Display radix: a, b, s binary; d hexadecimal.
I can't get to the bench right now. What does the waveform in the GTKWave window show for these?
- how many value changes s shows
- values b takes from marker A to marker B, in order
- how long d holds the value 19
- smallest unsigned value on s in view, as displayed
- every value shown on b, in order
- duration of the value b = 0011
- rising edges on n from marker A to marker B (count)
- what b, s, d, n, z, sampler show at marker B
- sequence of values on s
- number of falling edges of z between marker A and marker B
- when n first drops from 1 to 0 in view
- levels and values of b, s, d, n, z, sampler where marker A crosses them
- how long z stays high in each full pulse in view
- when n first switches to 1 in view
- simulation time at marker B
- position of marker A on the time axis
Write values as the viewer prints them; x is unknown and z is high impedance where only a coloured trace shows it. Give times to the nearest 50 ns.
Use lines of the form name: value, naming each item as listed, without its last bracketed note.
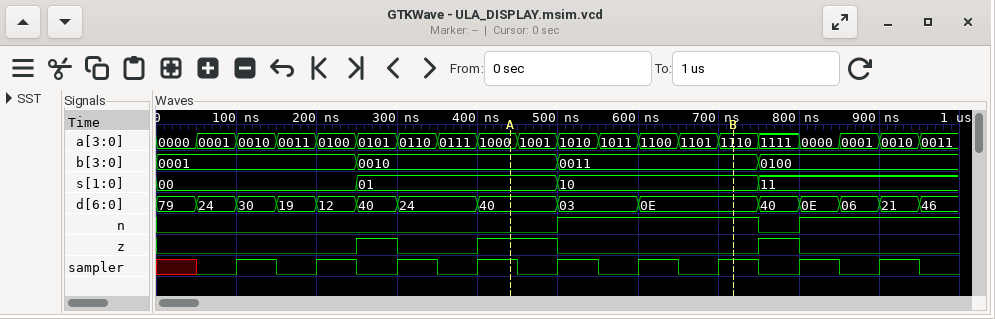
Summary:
how many value changes s shows: 3
values b takes from marker A to marker B, in order: 0010, 0011
how long d holds the value 19: 50 ns
smallest unsigned value on s in view, as displayed: 00
every value shown on b, in order: 0001, 0010, 0011, 0100
duration of the value b = 0011: 250 ns
rising edges on n from marker A to marker B: 1
what b, s, d, n, z, sampler show at marker B: b=0011, s=10, d=0E, n=1, z=0, sampler=1
sequence of values on s: 00, 01, 10, 11
number of falling edges of z between marker A and marker B: 1
when n first drops from 1 to 0 in view: 750 ns
levels and values of b, s, d, n, z, sampler where marker A crosses them: b=0010, s=01, d=40, n=0, z=1, sampler=1
how long z stays high in each full pulse in view: 50 ns, 100 ns, 50 ns
when n first switches to 1 in view: 500 ns
simulation time at marker B: 700 ns
position of marker A on the time axis: 450 ns
